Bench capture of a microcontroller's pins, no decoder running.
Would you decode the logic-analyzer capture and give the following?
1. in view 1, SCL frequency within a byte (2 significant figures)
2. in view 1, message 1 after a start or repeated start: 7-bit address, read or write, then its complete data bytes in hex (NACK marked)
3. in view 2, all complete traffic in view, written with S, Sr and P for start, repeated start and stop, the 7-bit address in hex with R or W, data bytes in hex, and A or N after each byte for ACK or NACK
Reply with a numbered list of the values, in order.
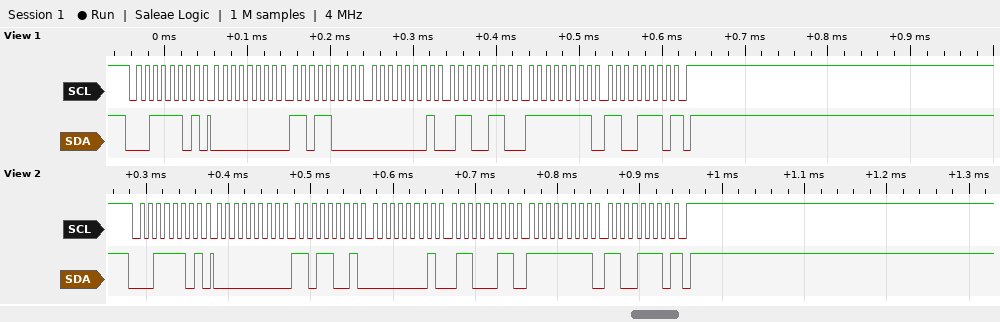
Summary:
1. 100 kHz
2. 0x1E read: 00 D8 01 66 FF CE NACK
3. S 1ER A 00 A D9 A 01 A 63 A FF A CE N P
